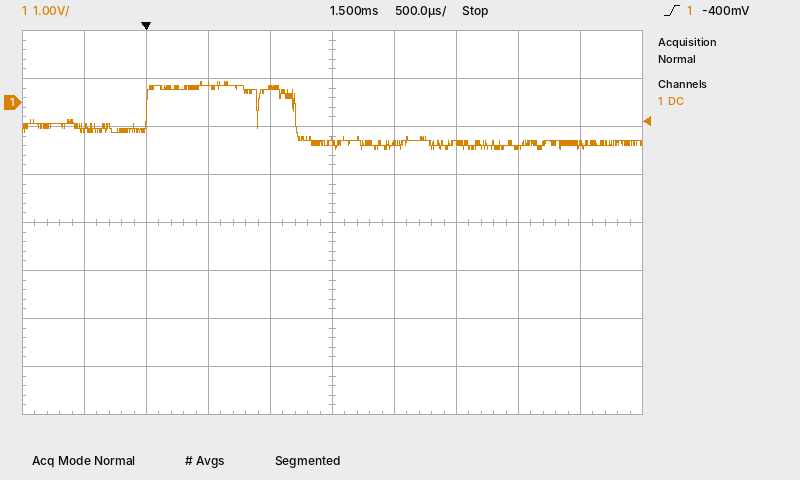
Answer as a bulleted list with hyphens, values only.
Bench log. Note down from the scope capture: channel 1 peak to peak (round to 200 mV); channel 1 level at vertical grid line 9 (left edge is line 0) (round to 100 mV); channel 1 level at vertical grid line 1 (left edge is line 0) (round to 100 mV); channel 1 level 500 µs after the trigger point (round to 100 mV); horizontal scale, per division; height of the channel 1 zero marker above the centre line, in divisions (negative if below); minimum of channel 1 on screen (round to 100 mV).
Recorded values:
- 1.4 V
- -900 mV
- -500 mV
- 400 mV
- 500 µs
- +2.5 div
- -1.0 V
